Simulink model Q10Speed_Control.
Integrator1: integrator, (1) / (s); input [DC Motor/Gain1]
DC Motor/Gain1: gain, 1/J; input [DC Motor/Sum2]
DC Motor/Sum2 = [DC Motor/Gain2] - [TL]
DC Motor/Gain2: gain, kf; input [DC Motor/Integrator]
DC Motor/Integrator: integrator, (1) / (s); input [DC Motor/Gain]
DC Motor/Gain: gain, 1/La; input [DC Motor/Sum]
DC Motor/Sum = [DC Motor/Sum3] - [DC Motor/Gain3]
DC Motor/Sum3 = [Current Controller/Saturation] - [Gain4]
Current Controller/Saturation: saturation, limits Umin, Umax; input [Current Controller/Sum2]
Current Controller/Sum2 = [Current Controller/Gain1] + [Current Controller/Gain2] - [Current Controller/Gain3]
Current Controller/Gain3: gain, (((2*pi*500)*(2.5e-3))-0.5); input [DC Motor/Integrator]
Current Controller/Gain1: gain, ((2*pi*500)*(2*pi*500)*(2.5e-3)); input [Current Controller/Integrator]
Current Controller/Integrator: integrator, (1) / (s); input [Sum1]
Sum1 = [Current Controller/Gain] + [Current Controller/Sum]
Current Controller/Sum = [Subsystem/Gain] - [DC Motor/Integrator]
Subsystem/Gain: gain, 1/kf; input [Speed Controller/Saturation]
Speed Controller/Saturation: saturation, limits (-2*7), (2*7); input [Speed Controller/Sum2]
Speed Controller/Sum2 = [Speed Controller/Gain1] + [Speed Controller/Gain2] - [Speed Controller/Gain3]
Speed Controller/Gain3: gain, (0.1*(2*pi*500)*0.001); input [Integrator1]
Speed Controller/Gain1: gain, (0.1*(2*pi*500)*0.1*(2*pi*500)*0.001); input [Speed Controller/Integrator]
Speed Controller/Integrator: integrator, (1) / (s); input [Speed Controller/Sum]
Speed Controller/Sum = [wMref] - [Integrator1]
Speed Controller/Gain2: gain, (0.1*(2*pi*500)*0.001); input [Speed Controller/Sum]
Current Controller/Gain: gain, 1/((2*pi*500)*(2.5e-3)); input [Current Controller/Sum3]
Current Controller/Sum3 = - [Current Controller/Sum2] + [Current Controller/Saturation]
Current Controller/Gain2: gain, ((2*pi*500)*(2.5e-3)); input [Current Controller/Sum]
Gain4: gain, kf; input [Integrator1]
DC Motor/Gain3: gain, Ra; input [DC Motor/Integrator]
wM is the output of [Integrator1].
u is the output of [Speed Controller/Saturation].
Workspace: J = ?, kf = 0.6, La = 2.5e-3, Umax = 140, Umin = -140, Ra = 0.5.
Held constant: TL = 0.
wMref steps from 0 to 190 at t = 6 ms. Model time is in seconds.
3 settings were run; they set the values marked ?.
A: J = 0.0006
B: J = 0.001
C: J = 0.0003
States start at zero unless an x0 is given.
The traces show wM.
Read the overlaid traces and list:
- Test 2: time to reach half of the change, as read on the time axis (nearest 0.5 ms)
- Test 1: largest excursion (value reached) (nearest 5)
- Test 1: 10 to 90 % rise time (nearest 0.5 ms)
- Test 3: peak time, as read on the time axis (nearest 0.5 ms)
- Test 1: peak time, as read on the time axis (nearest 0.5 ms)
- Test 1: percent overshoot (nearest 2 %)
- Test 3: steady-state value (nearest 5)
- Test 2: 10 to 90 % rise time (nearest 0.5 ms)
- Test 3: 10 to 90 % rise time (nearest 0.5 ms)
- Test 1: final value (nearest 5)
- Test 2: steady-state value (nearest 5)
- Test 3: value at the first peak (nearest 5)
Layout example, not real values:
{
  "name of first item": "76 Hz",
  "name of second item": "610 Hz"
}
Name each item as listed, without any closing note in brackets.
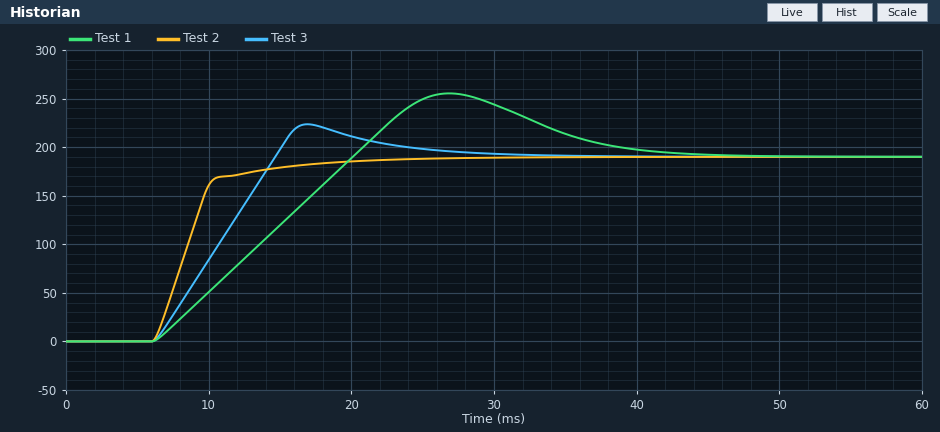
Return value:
{
  "Test 2: time to reach half of the change, as read on the time axis": "8.5 ms",
  "Test 1: largest excursion (value reached)": "255",
  "Test 1: 10 to 90 % rise time": "11.0 ms",
  "Test 3: peak time, as read on the time axis": "17.0 ms",
  "Test 1: peak time, as read on the time axis": "27.0 ms",
  "Test 1: percent overshoot": "34 %",
  "Test 3: steady-state value": "190",
  "Test 2: 10 to 90 % rise time": "5.0 ms",
  "Test 3: 10 to 90 % rise time": "6.5 ms",
  "Test 1: final value": "190",
  "Test 2: steady-state value": "190",
  "Test 3: value at the first peak": "225"
}
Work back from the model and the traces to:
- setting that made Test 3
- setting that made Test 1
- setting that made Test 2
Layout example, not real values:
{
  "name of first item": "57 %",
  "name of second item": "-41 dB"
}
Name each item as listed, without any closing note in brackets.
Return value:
{
  "setting that made Test 3": "A",
  "setting that made Test 1": "B",
  "setting that made Test 2": "C"
}
